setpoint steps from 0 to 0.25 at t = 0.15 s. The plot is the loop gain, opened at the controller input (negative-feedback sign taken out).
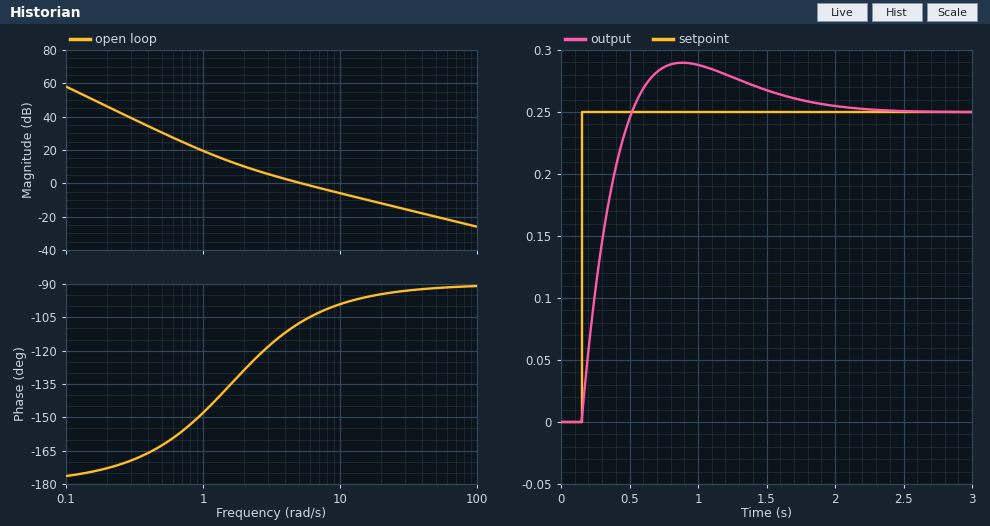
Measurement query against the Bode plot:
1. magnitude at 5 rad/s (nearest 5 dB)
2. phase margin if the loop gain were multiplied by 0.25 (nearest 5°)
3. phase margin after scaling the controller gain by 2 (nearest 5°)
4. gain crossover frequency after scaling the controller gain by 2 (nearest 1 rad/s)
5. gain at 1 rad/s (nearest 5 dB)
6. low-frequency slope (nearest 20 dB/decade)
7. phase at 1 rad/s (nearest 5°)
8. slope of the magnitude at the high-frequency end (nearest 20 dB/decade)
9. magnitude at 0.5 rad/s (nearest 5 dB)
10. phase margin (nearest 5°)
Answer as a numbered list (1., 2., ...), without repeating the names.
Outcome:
1. 0 dB
2. 45°
3. 80°
4. 10 rad/s
5. 20 dB
6. -40 dB/decade
7. -150°
8. -20 dB/decade
9. 30 dB
10. 75°
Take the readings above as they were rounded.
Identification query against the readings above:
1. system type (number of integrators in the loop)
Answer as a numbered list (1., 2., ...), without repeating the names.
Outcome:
1. 2
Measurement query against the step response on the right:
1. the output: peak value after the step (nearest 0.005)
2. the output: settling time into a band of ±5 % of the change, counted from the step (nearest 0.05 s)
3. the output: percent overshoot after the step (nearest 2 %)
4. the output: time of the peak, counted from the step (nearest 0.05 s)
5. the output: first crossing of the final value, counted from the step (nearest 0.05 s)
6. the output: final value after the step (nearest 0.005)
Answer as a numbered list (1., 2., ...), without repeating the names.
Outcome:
1. 0.290
2. 1.50 s
3. 16 %
4. 0.75 s
5. 0.35 s
6. 0.250
